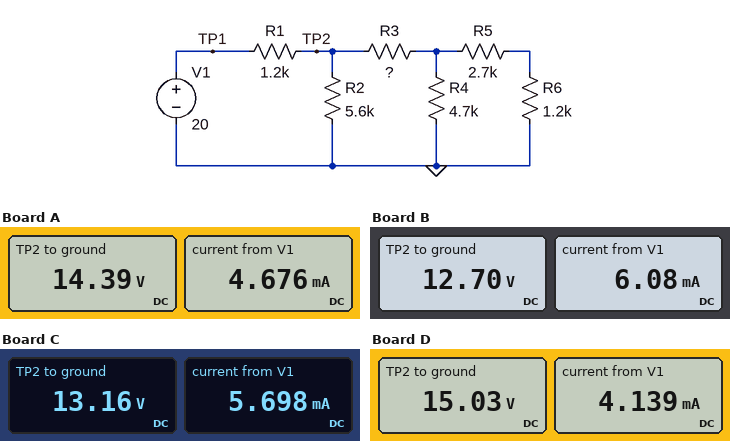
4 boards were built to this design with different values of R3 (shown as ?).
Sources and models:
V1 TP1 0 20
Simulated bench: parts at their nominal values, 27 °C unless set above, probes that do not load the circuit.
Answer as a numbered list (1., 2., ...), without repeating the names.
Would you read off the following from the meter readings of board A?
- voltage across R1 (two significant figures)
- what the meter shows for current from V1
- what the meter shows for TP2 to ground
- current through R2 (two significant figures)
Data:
1. 5.6 V
2. 4.676 mA
3. 14.39 V
4. 2.6 mA
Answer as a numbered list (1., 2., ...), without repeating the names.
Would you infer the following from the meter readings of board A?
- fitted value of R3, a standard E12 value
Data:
1. 4.7 kΩ
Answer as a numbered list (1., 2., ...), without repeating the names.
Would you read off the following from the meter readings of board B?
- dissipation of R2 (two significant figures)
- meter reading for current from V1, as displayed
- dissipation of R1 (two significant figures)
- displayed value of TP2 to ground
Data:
1. 29 mW
2. 6.08 mA
3. 44 mW
4. 12.70 V
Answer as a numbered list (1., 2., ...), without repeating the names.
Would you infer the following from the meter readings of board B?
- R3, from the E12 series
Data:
1. 1.2 kΩ
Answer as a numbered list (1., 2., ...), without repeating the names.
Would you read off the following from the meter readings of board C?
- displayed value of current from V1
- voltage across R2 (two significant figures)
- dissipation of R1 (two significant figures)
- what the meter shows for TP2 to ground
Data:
1. 5.698 mA
2. 13 V
3. 39 mW
4. 13.16 V
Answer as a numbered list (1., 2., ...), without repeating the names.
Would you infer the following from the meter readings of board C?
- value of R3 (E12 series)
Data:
1. 1.8 kΩ
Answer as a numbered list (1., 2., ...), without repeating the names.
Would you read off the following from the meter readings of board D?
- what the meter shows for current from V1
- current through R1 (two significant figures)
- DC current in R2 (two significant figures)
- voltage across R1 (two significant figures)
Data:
1. 4.139 mA
2. 4.1 mA
3. 2.7 mA
4. 5.0 V
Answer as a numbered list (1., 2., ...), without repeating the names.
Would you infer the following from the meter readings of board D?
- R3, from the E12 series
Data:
1. 8.2 kΩ
